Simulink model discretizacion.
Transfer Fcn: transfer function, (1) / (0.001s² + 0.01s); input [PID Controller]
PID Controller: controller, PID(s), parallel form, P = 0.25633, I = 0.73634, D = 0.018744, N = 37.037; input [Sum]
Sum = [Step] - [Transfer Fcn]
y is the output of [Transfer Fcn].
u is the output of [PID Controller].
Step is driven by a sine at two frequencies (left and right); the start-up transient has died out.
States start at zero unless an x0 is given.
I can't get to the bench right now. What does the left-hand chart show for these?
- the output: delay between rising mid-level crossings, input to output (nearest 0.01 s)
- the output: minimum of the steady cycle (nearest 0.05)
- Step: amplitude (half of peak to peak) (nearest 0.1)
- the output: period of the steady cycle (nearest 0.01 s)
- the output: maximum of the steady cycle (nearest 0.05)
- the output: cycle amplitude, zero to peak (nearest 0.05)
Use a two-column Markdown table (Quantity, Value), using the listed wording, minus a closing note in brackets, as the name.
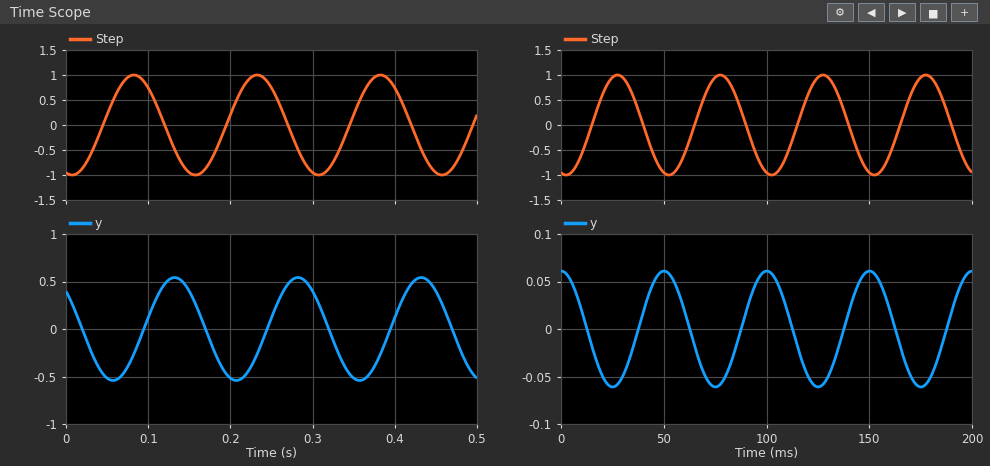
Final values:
| Quantity | Value |
|---|---|
| the output: delay between rising mid-level crossings, input to output | 0.05 s |
| the output: minimum of the steady cycle | -0.55 |
| Step: amplitude (half of peak to peak) | 1.0 |
| the output: period of the steady cycle | 0.15 s |
| the output: maximum of the steady cycle | 0.55 |
| the output: cycle amplitude, zero to peak | 0.55 |
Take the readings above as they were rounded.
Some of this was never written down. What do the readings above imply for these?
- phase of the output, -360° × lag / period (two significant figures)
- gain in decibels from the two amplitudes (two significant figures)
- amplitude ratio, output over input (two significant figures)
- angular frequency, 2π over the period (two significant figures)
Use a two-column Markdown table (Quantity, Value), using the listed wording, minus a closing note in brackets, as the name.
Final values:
| Quantity | Value |
|---|---|
| phase of the output, -360° × lag / period | -120° |
| gain in decibels from the two amplitudes | -5.2 dB |
| amplitude ratio, output over input | 0.55 |
| angular frequency, 2π over the period | 42 rad/s |
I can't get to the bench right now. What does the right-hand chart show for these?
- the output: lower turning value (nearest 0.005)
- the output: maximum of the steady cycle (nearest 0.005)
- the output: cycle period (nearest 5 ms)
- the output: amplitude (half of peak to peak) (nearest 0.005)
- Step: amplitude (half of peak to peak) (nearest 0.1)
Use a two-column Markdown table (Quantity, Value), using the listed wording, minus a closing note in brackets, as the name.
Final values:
| Quantity | Value |
|---|---|
| the output: lower turning value | -0.060 |
| the output: maximum of the steady cycle | 0.060 |
| the output: cycle period | 50 ms |
| the output: amplitude (half of peak to peak) | 0.060 |
| Step: amplitude (half of peak to peak) | 1.0 |
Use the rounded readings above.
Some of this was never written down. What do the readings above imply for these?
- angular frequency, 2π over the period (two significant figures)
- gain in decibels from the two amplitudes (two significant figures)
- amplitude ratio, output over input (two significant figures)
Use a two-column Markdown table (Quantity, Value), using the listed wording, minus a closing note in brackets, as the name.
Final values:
| Quantity | Value |
|---|---|
| angular frequency, 2π over the period | 0.13 rad/ms |
| gain in decibels from the two amplitudes | -24 dB |
| amplitude ratio, output over input | 0.060 |
